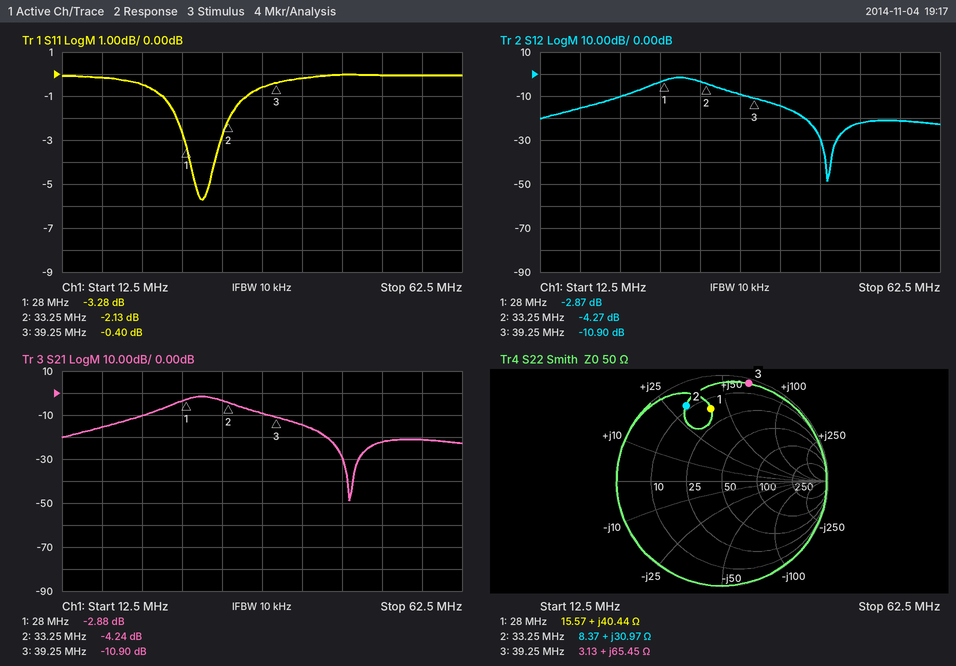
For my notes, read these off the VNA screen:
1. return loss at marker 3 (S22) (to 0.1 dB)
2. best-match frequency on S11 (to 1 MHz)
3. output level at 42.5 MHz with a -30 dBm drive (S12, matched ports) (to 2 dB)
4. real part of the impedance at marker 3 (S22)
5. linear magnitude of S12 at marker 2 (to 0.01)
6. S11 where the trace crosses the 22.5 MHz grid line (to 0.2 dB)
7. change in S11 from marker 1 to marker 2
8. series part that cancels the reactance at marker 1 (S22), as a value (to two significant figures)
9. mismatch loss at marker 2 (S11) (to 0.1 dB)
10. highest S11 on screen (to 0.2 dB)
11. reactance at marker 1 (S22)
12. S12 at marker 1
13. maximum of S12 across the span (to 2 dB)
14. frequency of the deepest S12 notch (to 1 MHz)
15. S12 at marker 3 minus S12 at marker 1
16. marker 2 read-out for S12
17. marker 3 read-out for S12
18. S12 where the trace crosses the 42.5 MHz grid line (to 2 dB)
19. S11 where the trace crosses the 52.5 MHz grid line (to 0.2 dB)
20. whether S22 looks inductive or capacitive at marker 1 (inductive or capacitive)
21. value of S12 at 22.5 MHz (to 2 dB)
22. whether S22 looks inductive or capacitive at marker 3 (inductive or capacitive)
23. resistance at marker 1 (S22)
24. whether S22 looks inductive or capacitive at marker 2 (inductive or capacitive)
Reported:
0.4 dB
30 MHz
-44 dBm
3.13 Ω
0.61
-0.4 dB
1.15 dB
140 pF
4.1 dB
0.0 dB
+40.44 Ω
-2.87 dB
-2 dB
48 MHz
-8.03 dB
-4.27 dB
-10.90 dB
-14 dB
0.0 dB
inductive
-10 dB
inductive
15.57 Ω
inductive
